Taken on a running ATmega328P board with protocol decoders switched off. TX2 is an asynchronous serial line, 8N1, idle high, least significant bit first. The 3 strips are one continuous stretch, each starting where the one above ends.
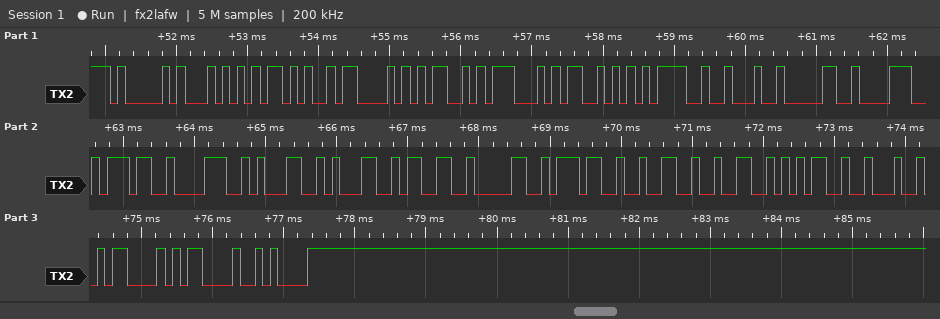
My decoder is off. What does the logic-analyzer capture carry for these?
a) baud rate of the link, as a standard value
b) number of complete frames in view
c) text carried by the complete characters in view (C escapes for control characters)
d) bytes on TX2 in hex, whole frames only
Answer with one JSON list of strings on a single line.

["9600 baud", "25", "\"AT+CMGS=\\\"087811307225\\\"\\r\\r\\n\"", "41 54 2B 43 4D 47 53 3D 22 30 38 37 38 31 31 33 30 37 32 32 35 22 0D 0D 0A"]
